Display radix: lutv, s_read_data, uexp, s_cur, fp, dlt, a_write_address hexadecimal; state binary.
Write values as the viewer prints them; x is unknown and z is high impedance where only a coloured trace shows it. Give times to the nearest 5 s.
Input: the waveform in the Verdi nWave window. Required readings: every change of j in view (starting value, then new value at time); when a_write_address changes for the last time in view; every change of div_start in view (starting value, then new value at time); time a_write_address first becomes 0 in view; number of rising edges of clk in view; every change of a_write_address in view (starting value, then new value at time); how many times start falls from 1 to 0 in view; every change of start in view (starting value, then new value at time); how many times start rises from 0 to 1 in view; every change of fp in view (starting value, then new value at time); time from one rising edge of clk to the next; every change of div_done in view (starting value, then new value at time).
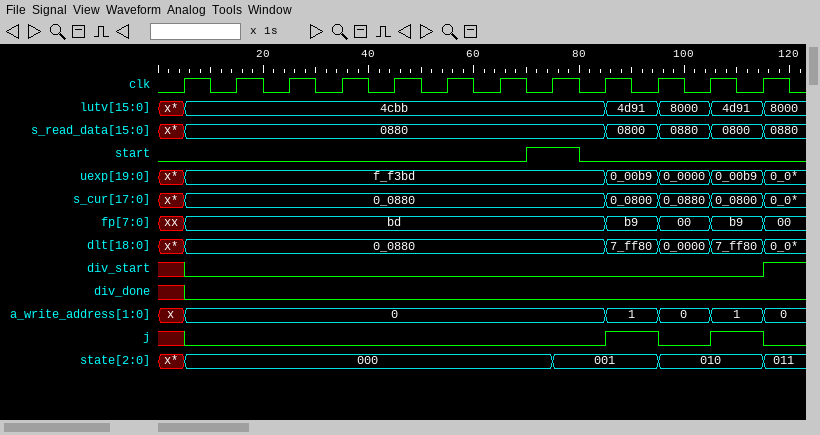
x, 0 at 5 s, 1 at 85 s, 0 at 95 s, 1 at 105 s, 0 at 115 s
115 s
x, 0 at 5 s, 1 at 115 s
5 s
12
x, 0 at 5 s, 1 at 85 s, 0 at 95 s, 1 at 105 s, 0 at 115 s
1
0, 1 at 70 s, 0 at 80 s
1
xx, bd at 5 s, b9 at 85 s, 00 at 95 s, b9 at 105 s, 00 at 115 s
10 s
x, 0 at 5 s
